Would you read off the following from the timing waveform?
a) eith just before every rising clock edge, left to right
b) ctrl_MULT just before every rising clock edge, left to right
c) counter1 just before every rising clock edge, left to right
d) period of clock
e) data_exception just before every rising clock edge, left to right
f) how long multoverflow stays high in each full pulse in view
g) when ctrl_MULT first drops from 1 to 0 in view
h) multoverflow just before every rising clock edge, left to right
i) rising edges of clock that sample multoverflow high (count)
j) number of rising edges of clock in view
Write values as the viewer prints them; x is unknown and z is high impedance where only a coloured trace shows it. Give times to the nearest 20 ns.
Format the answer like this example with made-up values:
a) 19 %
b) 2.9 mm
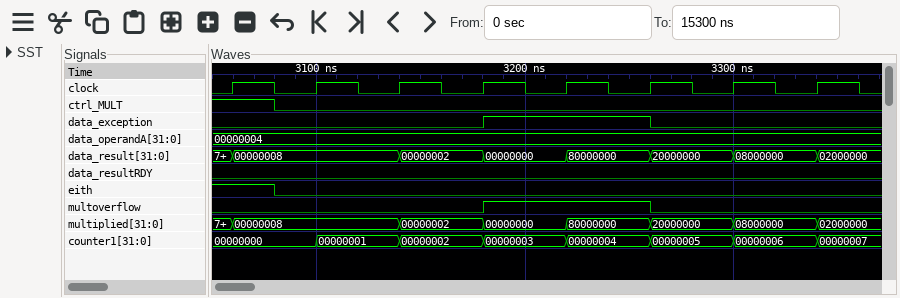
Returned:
a) 1 0 0 0 0 0 0 0
b) 1 0 0 0 0 0 0 0
c) 00000000, 00000000, 00000001, 00000002, 00000003, 00000004, 00000005, 00000006
d) 40 ns
e) 0 0 0 0 1 1 0 0
f) 80 ns
g) 3080 ns
h) 0 0 0 0 1 1 0 0
i) 2
j) 8
